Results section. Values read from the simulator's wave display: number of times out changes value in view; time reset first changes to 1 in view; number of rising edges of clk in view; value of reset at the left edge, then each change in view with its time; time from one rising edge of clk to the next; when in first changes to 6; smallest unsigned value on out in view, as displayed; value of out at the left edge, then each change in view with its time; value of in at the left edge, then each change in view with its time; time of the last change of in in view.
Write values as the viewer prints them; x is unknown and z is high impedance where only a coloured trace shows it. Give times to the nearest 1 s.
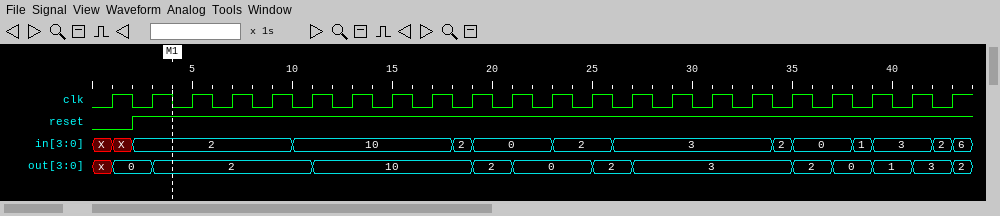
12
2 s
22
0, 1 at 2 s
2 s
43 s
0
x, 0 at 1 s, 2 at 3 s, 10 at 11 s, 2 at 19 s, 0 at 21 s, 2 at 25 s, 3 at 27 s, 2 at 35 s, 0 at 37 s, 1 at 39 s, 3 at 41 s, 2 at 43 s
X, X at 1 s, 2 at 2 s, 10 at 10 s, 2 at 18 s, 0 at 19 s, 2 at 23 s, 3 at 26 s, 2 at 34 s, 0 at 35 s, 1 at 38 s, 3 at 39 s, 2 at 42 s, 6 at 43 s
43 s
